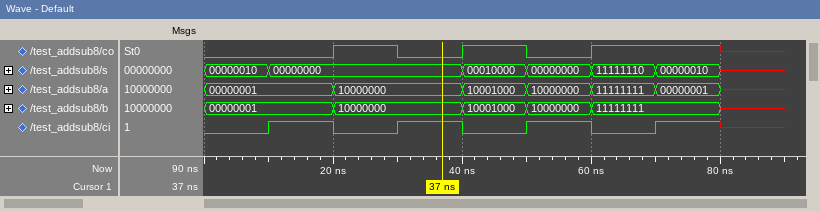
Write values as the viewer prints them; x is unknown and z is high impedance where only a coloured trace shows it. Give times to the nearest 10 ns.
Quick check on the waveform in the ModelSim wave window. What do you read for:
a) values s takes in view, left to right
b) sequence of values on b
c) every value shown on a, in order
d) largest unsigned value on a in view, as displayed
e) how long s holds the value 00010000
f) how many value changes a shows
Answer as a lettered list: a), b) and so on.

a) 00000010, 00000000, 00010000, 00000000, 11111110, 00000010, x
b) 00000001, 10000000, 10001000, 10000000, 11111111, x
c) 00000001, 10000000, 10001000, 10000000, 11111111, 00000001, x
d) 11111111
e) 10 ns
f) 6
